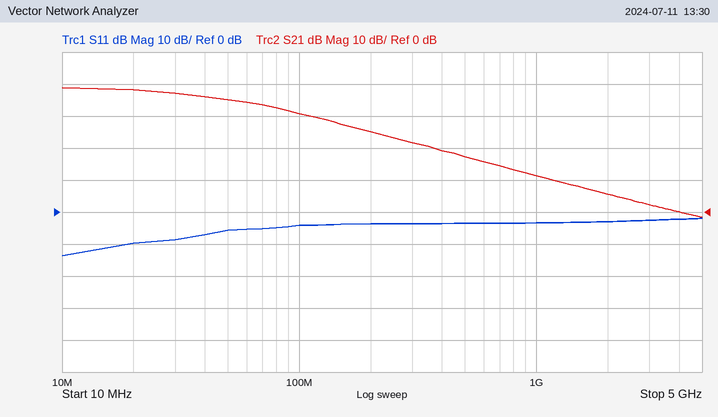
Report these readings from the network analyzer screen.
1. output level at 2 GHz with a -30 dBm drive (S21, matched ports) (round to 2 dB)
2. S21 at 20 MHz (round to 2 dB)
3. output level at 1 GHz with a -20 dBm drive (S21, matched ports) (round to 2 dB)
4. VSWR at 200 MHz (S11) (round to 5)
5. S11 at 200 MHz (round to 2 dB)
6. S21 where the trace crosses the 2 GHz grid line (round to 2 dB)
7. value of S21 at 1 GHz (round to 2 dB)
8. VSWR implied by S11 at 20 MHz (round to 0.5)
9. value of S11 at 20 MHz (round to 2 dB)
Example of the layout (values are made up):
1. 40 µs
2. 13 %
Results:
1. -24 dBm
2. 38 dB
3. -8 dBm
4. 5
5. -4 dB
6. 6 dB
7. 12 dB
8. 2.0
9. -10 dB
